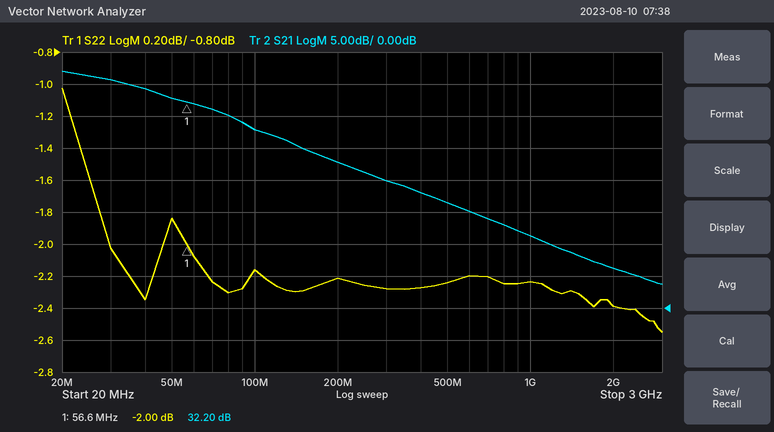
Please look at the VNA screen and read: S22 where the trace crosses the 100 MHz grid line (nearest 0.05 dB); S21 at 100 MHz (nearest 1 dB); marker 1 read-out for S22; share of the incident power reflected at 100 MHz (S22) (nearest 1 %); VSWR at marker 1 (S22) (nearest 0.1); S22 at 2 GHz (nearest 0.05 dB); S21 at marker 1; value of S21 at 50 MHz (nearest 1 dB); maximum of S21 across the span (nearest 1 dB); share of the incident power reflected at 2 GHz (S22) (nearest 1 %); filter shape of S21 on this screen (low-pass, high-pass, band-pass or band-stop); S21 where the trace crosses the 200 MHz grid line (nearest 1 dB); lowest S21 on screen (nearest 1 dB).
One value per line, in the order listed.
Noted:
-2.15 dB
28 dB
-2.00 dB
61 %
8.7
-2.40 dB
32.20 dB
33 dB
37 dB
58 %
low-pass
23 dB
4 dB
